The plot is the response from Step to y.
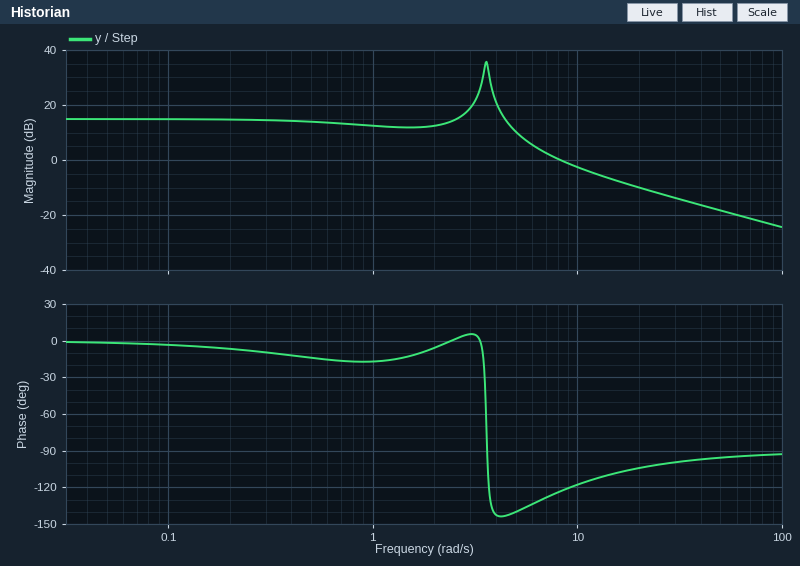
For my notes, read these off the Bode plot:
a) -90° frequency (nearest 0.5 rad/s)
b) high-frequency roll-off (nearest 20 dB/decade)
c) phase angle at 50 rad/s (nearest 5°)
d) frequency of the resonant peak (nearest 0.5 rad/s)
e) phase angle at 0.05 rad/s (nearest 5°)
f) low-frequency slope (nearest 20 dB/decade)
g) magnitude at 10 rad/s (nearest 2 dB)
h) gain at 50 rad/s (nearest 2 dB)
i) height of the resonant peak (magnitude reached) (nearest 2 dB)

3.5 rad/s
-20 dB/decade
-95°
3.5 rad/s
0°
0 dB/decade
-2 dB
-18 dB
36 dB
